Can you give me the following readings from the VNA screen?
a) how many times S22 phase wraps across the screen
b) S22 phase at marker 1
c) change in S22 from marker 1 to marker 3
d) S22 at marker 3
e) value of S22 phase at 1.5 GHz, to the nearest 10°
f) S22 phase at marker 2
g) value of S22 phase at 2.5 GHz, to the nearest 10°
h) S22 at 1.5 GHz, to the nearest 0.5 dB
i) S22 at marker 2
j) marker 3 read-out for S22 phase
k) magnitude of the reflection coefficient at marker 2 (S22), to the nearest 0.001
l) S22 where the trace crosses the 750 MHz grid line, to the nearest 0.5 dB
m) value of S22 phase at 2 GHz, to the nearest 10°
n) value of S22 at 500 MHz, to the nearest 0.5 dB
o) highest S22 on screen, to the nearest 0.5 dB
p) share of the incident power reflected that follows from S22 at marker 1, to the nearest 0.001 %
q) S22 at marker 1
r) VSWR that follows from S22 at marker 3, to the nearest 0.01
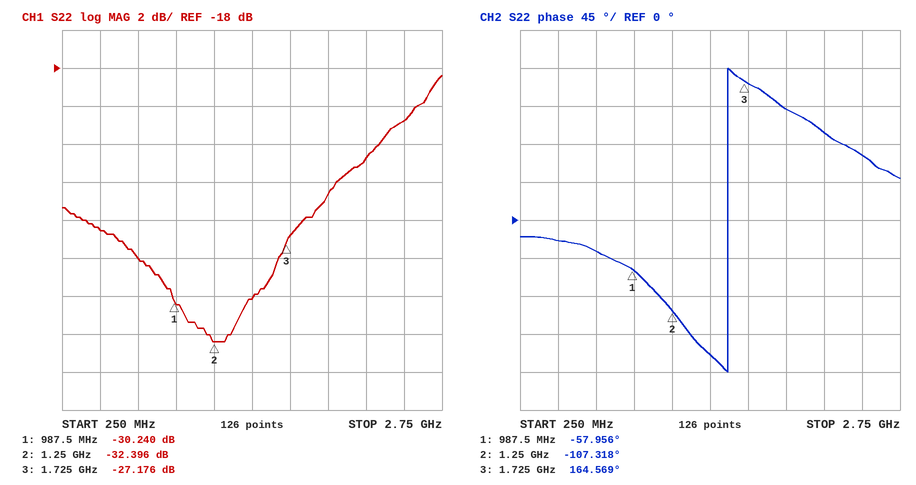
1
-57.956°
3.064 dB
-27.176 dB
-160°
-107.318°
80°
-30.0 dB
-32.396 dB
164.569°
0.024
-28.0 dB
130°
-26.5 dB
-18.5 dB
0.095 %
-30.240 dB
1.09
